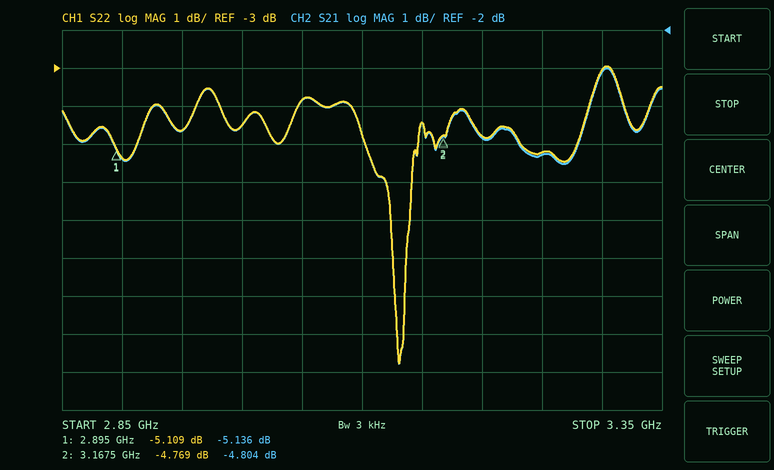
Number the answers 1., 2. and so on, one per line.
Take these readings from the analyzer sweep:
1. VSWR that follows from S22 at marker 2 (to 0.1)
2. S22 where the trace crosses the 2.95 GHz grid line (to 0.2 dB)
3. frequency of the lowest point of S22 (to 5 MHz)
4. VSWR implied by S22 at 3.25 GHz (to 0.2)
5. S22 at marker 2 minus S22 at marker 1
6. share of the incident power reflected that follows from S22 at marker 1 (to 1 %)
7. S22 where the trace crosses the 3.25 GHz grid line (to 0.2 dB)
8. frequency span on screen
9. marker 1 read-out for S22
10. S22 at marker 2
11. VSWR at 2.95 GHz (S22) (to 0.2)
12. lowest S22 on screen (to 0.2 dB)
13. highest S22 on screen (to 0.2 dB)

1. 3.7
2. -4.6 dB
3. 3.130 GHz
4. 3.4
5. 0.340 dB
6. 31 %
7. -5.2 dB
8. 500 MHz
9. -5.109 dB
10. -4.769 dB
11. 3.8
12. -10.8 dB
13. -3.0 dB
